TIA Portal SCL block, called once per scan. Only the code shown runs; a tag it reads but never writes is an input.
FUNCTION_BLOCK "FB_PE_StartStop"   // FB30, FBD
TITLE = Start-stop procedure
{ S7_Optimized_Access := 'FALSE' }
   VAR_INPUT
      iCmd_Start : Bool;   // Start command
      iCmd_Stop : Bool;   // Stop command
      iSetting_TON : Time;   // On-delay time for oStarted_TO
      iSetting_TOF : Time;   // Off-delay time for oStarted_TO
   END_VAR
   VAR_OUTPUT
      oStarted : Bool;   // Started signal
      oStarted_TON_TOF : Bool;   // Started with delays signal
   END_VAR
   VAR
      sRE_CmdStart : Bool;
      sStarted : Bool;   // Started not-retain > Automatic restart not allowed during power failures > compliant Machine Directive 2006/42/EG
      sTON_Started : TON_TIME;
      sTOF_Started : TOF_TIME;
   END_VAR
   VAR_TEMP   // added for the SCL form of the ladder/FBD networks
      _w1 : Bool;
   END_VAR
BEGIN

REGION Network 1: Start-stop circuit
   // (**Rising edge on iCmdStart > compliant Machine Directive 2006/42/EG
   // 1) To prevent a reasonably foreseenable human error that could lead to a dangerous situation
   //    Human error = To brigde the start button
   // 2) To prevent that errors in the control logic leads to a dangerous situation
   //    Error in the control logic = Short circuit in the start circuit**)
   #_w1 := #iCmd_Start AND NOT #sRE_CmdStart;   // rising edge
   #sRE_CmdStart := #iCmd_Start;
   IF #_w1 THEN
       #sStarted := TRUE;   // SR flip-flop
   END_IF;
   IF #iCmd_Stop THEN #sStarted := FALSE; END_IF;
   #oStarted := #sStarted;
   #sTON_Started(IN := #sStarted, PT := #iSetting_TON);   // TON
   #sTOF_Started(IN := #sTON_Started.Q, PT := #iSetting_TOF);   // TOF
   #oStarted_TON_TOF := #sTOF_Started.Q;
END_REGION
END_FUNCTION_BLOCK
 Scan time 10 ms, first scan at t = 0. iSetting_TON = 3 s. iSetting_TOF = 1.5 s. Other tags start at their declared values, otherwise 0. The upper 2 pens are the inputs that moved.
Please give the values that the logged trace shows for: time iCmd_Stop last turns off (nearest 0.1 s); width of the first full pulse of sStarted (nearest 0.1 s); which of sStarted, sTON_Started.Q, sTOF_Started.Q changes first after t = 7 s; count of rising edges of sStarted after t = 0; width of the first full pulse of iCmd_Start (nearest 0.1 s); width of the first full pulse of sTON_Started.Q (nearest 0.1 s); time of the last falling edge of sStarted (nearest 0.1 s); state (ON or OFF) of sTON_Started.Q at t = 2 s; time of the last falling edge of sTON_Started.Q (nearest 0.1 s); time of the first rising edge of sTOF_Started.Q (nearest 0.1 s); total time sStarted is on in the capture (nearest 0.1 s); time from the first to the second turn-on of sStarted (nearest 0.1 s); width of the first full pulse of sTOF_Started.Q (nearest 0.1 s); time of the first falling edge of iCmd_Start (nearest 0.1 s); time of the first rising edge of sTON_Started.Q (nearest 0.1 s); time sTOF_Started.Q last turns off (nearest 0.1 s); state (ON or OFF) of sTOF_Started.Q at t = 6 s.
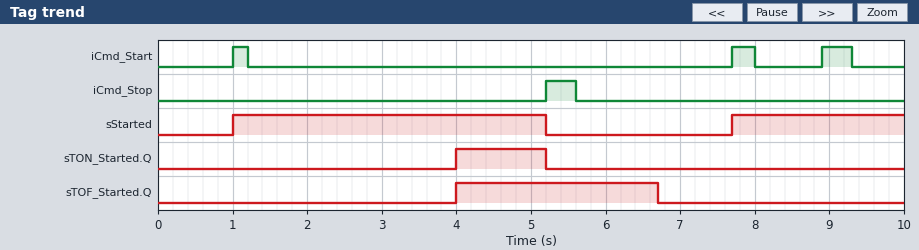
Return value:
5.6 s
4.2 s
sStarted
2
0.2 s
1.2 s
5.2 s
OFF
5.2 s
4.0 s
6.5 s
6.7 s
2.7 s
1.2 s
4.0 s
6.7 s
ON
